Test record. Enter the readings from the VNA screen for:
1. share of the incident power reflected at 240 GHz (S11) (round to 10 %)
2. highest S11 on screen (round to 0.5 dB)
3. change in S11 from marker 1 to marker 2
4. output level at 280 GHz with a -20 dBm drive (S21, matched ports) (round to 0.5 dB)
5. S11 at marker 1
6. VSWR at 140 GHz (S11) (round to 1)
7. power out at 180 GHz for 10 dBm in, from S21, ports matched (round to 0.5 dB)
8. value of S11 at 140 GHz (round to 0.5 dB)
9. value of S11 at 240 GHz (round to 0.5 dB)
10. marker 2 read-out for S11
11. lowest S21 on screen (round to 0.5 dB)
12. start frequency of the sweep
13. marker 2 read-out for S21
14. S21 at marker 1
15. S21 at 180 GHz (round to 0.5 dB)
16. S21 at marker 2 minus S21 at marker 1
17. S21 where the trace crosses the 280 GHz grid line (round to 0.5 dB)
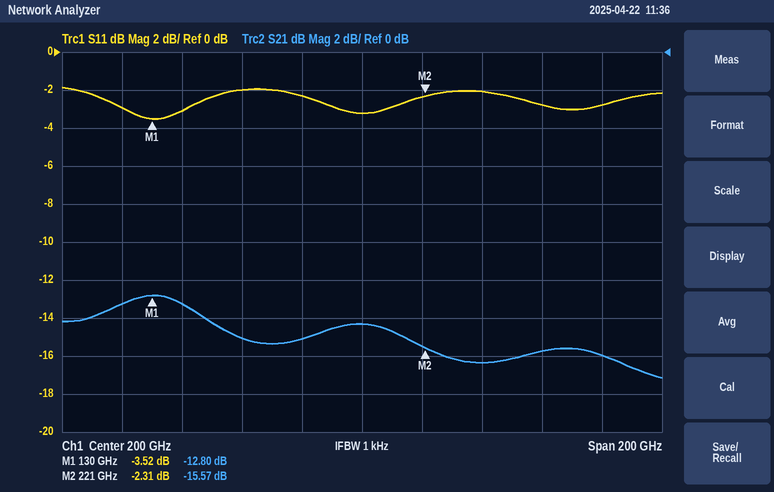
60 %
-2.0 dB
1.21 dB
-36.0 dBm
-3.52 dB
6
-5.0 dBm
-3.0 dB
-2.0 dB
-2.31 dB
-17.0 dB
100 GHz
-15.57 dB
-12.80 dB
-15.0 dB
-2.77 dB
-16.0 dB
